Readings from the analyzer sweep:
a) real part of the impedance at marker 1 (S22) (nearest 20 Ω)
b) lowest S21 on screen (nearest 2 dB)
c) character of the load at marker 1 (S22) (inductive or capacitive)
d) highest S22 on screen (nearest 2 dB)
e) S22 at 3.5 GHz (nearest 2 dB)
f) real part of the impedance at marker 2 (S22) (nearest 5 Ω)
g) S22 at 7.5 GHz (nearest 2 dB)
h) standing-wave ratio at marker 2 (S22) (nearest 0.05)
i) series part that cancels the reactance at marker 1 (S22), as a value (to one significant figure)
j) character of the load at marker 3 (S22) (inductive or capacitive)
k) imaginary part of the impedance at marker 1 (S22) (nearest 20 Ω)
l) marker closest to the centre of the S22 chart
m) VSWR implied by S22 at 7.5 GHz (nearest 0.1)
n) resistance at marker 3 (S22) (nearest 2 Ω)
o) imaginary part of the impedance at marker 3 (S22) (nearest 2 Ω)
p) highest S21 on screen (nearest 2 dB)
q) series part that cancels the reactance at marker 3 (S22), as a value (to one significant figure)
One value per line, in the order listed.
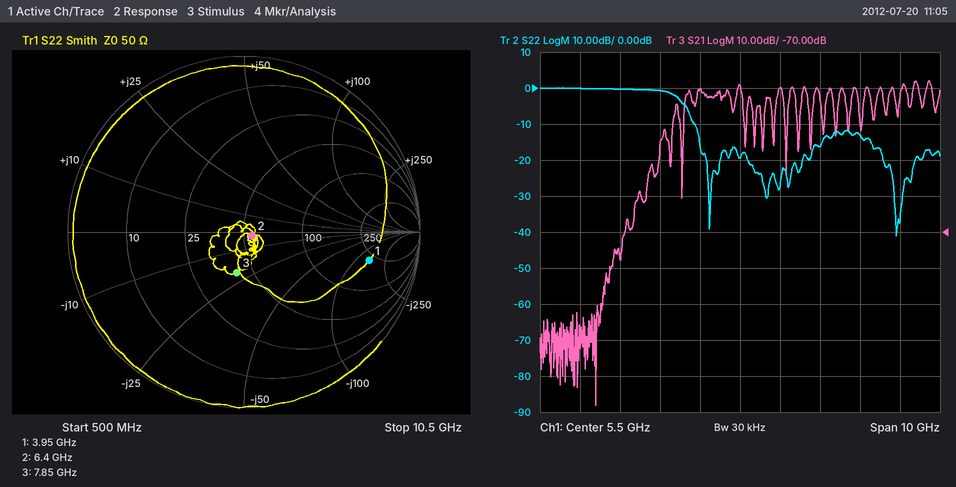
220 Ω
-118 dB
capacitive
0 dB
0 dB
55 Ω
-16 dB
1.10
6 nH
capacitive
-140 Ω
marker 2
1.4
42 Ω
-20 Ω
-28 dB
400 pH
